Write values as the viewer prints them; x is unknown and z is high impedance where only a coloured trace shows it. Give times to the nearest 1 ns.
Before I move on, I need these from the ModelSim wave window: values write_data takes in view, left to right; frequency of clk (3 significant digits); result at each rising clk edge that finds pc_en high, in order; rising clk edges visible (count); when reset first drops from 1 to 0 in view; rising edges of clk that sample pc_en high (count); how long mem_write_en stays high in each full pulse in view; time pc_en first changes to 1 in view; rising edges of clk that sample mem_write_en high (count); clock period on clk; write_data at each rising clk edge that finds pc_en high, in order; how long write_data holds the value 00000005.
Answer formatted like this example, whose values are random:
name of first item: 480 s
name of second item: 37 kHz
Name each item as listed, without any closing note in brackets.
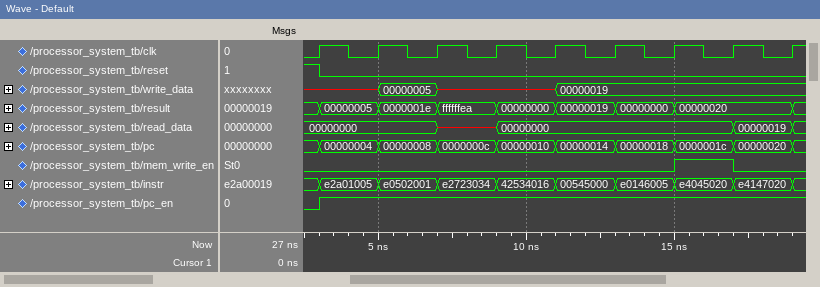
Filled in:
values write_data takes in view, left to right: x, 00000005, x, 00000019
frequency of clk: 500 MHz
result at each rising clk edge that finds pc_en high, in order: 00000005, 0000001e, ffffffea, 00000000, 00000019, 00000000, 00000020, 00000020
rising clk edges visible: 9
when reset first drops from 1 to 0 in view: 3 ns
rising edges of clk that sample pc_en high: 8
how long mem_write_en stays high in each full pulse in view: 2 ns
time pc_en first changes to 1 in view: 3 ns
rising edges of clk that sample mem_write_en high: 1
clock period on clk: 2 ns
write_data at each rising clk edge that finds pc_en high, in order: x, 00000005, x, x, 00000019, 00000019, 00000019, 00000019
how long write_data holds the value 00000005: 2 ns
